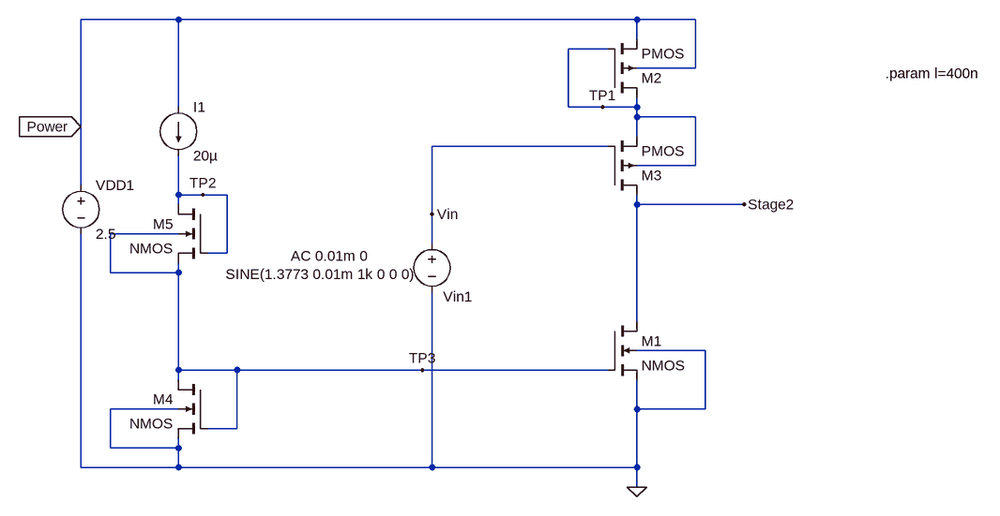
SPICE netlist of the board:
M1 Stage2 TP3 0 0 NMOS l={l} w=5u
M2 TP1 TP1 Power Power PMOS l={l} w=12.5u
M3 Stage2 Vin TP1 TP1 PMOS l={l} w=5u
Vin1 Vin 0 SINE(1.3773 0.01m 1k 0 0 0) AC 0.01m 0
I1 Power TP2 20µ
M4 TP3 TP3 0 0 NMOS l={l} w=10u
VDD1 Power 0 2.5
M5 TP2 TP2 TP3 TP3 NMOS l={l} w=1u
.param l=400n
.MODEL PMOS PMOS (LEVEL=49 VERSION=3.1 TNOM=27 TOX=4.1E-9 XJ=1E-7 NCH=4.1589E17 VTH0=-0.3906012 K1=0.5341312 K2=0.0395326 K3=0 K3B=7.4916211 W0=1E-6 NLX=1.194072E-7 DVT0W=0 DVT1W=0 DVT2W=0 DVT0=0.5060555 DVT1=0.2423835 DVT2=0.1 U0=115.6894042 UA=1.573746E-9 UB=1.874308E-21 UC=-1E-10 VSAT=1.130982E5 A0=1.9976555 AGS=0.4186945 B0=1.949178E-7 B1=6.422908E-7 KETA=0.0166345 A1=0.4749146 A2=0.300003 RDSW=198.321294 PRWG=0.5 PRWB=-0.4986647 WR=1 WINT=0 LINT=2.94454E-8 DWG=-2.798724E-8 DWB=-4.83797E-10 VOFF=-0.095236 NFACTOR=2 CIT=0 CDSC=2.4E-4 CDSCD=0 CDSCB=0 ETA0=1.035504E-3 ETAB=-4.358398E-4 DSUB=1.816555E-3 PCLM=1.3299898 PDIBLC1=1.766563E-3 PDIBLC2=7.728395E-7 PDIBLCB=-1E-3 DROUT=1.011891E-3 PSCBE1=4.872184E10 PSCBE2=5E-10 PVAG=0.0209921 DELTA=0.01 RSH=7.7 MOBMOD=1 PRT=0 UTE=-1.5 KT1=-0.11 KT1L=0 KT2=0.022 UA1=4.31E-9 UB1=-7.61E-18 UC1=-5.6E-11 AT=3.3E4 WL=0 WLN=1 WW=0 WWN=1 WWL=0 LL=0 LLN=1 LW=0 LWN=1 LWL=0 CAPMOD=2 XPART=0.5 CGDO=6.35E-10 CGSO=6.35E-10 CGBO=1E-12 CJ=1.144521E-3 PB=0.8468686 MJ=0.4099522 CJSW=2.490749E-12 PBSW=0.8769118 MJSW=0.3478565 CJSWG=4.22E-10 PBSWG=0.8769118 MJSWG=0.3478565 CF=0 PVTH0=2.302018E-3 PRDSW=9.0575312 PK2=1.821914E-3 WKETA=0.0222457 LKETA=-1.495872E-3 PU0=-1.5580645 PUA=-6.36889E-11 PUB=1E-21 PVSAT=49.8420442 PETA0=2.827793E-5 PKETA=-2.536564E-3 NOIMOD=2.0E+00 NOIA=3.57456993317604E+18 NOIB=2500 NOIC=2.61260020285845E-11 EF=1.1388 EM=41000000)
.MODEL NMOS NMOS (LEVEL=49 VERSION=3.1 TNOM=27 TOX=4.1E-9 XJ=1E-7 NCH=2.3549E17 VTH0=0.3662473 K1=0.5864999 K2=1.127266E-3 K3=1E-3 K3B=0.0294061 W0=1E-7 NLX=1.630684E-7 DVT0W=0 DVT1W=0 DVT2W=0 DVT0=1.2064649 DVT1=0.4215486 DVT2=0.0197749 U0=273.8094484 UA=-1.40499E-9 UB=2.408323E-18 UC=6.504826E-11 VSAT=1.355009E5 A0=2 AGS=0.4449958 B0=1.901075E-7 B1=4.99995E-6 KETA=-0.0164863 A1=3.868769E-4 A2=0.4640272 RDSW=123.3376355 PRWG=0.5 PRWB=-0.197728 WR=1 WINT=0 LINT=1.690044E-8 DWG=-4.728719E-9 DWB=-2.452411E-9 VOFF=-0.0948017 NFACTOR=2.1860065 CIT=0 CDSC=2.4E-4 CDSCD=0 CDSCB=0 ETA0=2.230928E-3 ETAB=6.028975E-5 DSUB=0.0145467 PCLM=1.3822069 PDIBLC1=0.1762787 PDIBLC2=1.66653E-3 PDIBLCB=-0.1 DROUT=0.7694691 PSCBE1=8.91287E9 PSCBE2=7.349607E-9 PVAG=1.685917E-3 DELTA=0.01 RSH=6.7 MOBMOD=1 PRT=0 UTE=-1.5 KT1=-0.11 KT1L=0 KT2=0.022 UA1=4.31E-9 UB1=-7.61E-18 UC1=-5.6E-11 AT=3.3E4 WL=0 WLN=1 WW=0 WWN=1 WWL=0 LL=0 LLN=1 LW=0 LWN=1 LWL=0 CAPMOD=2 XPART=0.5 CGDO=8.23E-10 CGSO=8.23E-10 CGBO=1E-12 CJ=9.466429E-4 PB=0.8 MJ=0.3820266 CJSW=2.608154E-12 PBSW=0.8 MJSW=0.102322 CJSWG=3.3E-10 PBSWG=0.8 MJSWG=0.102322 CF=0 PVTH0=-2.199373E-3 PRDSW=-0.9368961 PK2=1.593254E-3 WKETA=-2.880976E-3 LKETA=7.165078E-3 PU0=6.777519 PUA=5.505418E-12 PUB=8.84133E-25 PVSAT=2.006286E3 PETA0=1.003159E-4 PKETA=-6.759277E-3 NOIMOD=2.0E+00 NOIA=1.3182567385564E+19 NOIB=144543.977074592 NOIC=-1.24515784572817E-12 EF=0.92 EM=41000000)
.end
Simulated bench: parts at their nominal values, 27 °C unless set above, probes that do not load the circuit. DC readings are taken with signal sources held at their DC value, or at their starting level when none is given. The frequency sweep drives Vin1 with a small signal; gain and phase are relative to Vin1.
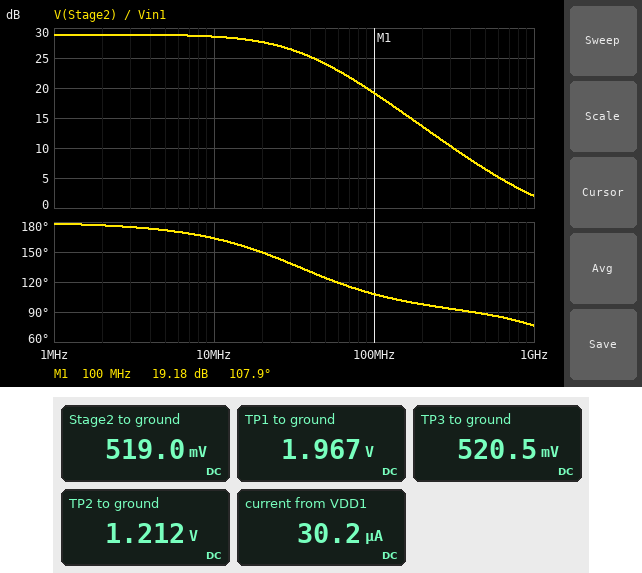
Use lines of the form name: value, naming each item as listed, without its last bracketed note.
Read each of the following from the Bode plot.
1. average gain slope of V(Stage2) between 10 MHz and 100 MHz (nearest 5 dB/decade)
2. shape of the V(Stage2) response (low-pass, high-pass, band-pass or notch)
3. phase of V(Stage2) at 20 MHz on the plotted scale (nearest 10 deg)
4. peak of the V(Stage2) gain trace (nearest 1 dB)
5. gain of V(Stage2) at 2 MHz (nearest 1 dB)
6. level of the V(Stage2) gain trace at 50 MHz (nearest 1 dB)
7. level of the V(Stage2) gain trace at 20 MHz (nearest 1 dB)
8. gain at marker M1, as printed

average gain slope of V(Stage2) between 10 MHz and 100 MHz: -10 dB/decade
shape of the V(Stage2) response: low-pass
phase of V(Stage2) at 20 MHz on the plotted scale: 150 deg
peak of the V(Stage2) gain trace: 29 dB
gain of V(Stage2) at 2 MHz: 29 dB
level of the V(Stage2) gain trace at 50 MHz: 24 dB
level of the V(Stage2) gain trace at 20 MHz: 28 dB
gain at marker M1, as printed: 19.18 dB
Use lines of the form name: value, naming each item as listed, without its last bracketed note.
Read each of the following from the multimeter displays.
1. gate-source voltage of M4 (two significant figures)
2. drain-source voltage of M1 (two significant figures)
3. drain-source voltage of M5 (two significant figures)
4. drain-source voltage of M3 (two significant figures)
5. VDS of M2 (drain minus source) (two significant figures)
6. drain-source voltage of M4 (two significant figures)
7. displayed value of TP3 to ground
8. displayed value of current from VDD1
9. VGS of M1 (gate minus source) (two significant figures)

gate-source voltage of M4: 520 mV
drain-source voltage of M1: 520 mV
drain-source voltage of M5: 690 mV
drain-source voltage of M3: -1.4 V
VDS of M2 (drain minus source): -530 mV
drain-source voltage of M4: 520 mV
displayed value of TP3 to ground: 520.5 mV
displayed value of current from VDD1: 30.2 µA
VGS of M1 (gate minus source): 520 mV
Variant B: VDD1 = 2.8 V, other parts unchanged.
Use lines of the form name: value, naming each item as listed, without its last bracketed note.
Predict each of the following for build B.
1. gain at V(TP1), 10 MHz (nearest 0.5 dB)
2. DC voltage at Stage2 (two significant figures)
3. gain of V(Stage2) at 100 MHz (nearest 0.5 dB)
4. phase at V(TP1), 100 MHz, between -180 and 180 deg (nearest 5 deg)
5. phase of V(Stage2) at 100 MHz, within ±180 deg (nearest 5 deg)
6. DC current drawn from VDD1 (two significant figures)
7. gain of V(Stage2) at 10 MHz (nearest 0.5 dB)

gain at V(TP1), 10 MHz: -43.5 dB
DC voltage at Stage2: 2.2 V
gain of V(Stage2) at 100 MHz: -18.5 dB
phase at V(TP1), 100 MHz, between -180 and 180 deg: 80 deg
phase of V(Stage2) at 100 MHz, within ±180 deg: 130 deg
DC current drawn from VDD1: 33 µA
gain of V(Stage2) at 10 MHz: -21.0 dB
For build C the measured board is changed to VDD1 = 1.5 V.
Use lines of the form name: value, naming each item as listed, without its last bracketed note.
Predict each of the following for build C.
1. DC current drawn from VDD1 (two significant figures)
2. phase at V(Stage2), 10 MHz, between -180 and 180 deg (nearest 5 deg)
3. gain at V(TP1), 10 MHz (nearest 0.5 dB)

DC current drawn from VDD1: 20 µA
phase at V(Stage2), 10 MHz, between -180 and 180 deg: 90 deg
gain at V(TP1), 10 MHz: -13.0 dB
